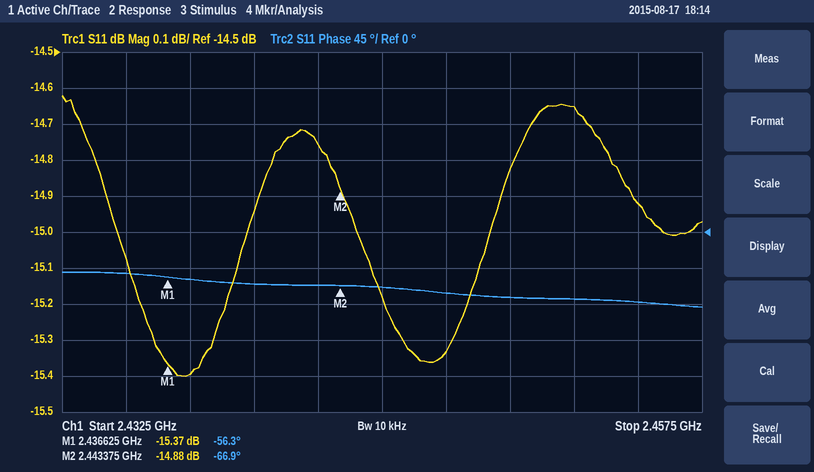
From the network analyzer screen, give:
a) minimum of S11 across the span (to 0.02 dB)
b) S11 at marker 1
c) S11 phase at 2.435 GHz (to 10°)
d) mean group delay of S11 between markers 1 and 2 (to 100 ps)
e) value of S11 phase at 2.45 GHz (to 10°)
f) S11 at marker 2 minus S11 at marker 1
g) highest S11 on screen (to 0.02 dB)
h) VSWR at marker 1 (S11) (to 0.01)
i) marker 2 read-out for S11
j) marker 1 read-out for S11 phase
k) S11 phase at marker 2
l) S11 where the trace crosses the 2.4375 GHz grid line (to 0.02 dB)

-15.40 dB
-15.37 dB
-50°
4.4 ns
-80°
0.49 dB
-14.62 dB
1.41
-14.88 dB
-56.3°
-66.9°
-15.40 dB
